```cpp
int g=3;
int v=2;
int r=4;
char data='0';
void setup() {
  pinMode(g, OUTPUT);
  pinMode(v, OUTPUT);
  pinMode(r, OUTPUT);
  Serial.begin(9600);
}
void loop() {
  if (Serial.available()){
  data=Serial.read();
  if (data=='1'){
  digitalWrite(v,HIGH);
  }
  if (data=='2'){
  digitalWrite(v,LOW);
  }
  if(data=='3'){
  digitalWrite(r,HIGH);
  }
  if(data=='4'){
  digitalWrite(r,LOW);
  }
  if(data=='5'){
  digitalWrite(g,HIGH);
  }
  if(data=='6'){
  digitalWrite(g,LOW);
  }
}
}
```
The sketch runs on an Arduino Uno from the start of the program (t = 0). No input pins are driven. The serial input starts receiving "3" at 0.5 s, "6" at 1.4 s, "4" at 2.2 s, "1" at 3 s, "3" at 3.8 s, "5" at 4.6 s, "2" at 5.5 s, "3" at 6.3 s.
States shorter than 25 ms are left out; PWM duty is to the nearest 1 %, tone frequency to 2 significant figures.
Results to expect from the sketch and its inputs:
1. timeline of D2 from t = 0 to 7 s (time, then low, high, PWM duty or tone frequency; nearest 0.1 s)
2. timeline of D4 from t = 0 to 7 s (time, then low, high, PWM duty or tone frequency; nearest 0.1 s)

0 s low; 3 s high; 5.5 s low
0 s low; 0.5 s high; 2.2 s low; 3.8 s high
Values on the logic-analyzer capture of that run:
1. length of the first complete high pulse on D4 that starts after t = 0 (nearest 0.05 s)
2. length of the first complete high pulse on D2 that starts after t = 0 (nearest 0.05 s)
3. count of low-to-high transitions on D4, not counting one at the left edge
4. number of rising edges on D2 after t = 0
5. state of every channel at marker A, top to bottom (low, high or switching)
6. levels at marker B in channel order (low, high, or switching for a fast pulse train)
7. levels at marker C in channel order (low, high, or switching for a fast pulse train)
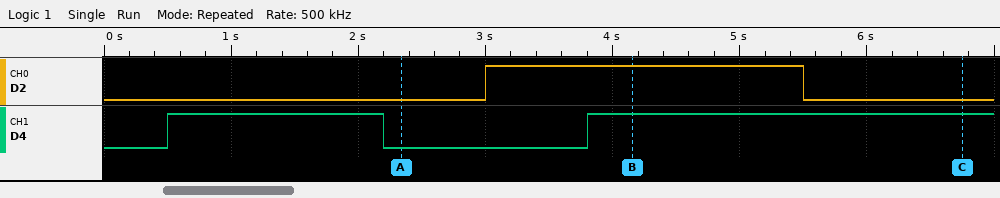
1.70 s
2.50 s
2
1
D2 low, D4 low
D2 high, D4 high
D2 low, D4 high
